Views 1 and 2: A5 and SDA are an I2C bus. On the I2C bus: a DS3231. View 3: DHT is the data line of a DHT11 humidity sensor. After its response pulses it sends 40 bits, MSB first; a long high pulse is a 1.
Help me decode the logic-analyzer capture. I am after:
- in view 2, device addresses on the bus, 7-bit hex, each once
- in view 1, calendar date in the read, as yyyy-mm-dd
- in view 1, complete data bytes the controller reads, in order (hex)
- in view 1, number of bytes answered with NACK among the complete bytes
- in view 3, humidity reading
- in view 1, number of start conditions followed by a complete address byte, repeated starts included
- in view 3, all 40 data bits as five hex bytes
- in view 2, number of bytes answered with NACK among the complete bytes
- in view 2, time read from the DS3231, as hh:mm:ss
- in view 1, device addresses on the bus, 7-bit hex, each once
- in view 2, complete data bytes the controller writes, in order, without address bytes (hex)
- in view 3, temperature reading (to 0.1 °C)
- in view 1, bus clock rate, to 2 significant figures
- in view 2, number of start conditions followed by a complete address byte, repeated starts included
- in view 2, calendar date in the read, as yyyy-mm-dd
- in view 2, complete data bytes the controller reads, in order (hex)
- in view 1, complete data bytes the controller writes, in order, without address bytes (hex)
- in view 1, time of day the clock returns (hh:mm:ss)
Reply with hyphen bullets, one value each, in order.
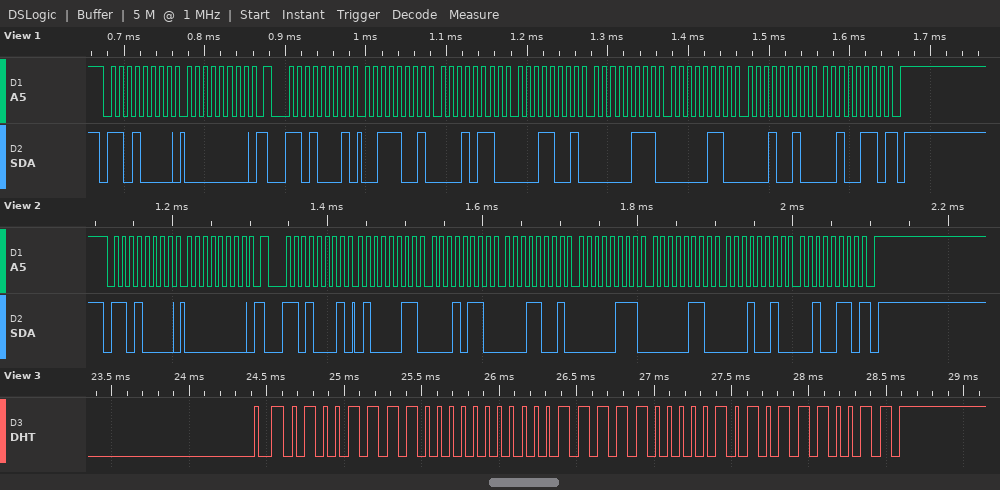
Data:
- 0x68
- 2026-12-06
- 39 16 19 07 06 12 26
- 1
- 79 %
- 2
- 4F 00 1F 05 73
- 1
- 19:16:43
- 0x68
- 00
- 31.5 °C
- 100 kHz
- 2
- 2026-12-06
- 43 16 19 07 06 12 26
- 00
- 19:16:39
